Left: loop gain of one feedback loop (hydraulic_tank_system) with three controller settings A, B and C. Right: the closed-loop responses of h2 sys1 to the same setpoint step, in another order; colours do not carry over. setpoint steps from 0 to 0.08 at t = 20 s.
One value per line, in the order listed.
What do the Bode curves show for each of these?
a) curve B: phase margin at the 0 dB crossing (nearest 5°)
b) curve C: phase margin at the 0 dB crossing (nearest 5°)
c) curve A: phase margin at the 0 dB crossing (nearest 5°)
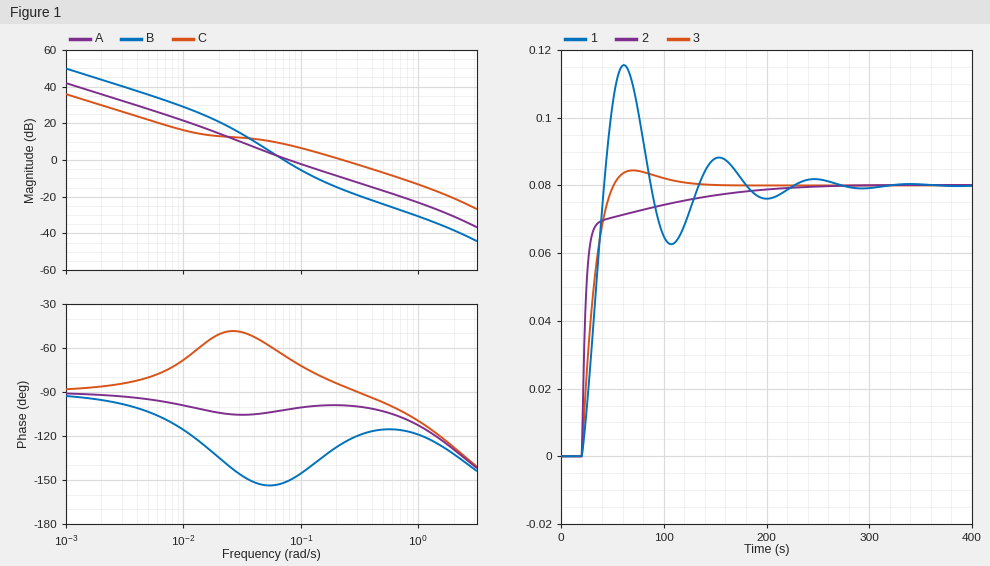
30°
95°
80°
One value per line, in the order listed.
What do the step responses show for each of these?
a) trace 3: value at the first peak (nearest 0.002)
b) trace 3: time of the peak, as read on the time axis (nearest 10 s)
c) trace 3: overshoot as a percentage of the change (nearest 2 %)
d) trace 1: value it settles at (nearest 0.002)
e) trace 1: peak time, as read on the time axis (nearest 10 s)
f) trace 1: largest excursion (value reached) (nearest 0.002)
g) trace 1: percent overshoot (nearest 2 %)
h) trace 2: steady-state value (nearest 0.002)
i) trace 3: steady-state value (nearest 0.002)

0.084
70 s
6 %
0.080
60 s
0.116
44 %
0.080
0.080
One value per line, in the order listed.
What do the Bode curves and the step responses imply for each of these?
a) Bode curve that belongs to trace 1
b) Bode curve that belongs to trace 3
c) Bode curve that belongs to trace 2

B
A
C
